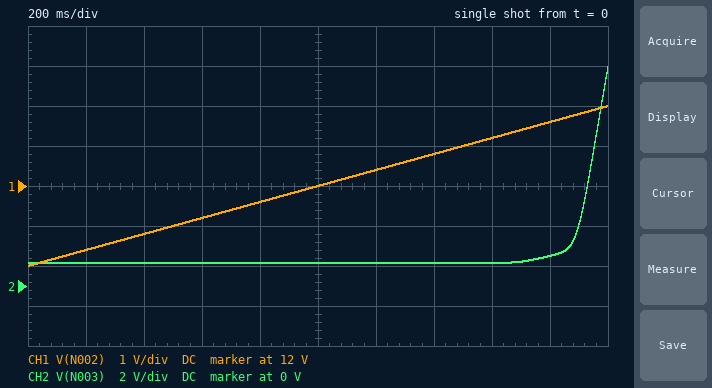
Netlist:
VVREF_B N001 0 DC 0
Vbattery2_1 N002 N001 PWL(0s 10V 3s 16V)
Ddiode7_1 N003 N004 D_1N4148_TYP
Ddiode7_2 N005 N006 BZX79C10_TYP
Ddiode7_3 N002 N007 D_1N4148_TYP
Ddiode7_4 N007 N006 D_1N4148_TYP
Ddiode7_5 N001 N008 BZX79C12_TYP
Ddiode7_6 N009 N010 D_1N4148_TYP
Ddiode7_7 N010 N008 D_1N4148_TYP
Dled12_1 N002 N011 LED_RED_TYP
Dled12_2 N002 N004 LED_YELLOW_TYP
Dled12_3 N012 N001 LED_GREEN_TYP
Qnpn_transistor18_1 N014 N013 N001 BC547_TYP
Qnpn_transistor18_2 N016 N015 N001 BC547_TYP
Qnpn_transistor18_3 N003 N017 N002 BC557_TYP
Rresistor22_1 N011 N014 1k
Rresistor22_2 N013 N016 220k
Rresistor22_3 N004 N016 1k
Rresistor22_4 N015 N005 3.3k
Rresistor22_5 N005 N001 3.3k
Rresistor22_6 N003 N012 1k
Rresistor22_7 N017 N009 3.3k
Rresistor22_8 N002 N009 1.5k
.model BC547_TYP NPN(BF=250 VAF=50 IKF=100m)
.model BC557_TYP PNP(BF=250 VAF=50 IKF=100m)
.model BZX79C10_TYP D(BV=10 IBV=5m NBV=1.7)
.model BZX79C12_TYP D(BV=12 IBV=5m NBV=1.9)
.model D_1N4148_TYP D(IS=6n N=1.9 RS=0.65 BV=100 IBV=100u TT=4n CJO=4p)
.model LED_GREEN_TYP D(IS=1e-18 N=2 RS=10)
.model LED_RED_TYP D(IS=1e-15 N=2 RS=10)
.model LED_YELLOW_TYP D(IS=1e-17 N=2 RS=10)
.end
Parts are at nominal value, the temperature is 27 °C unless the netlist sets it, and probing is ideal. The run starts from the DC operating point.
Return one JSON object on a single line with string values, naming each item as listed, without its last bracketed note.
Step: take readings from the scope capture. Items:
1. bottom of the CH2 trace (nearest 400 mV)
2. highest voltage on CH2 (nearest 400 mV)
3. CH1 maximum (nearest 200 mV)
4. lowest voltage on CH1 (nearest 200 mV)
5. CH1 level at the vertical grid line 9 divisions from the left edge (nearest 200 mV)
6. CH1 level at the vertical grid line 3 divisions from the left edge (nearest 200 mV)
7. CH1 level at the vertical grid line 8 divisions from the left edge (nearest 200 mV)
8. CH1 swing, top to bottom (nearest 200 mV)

{"bottom of the CH2 trace": "1.2 V", "highest voltage on CH2": "10.8 V", "CH1 maximum": "14.0 V", "lowest voltage on CH1": "10.0 V", "CH1 level at the vertical grid line 9 divisions from the left edge": "13.6 V", "CH1 level at the vertical grid line 3 divisions from the left edge": "11.2 V", "CH1 level at the vertical grid line 8 divisions from the left edge": "13.2 V", "CH1 swing, top to bottom": "4.0 V"}
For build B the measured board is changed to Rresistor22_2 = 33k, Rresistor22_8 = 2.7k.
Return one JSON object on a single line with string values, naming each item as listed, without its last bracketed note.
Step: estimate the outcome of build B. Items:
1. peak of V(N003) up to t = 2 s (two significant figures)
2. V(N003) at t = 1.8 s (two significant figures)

{"peak of V(N003) up to t = 2 s": "13 V", "V(N003) at t = 1.8 s": "1.7 V"}
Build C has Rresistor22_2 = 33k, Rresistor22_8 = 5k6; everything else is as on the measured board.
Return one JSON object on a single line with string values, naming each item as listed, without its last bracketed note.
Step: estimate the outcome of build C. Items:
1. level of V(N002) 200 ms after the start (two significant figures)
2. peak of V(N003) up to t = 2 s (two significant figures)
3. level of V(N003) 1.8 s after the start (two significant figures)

{"level of V(N002) 200 ms after the start": "10 V", "peak of V(N003) up to t = 2 s": "13 V", "level of V(N003) 1.8 s after the start": "2.9 V"}
